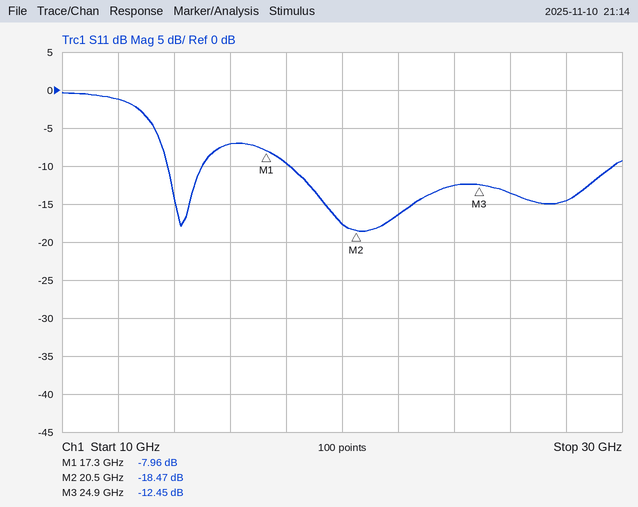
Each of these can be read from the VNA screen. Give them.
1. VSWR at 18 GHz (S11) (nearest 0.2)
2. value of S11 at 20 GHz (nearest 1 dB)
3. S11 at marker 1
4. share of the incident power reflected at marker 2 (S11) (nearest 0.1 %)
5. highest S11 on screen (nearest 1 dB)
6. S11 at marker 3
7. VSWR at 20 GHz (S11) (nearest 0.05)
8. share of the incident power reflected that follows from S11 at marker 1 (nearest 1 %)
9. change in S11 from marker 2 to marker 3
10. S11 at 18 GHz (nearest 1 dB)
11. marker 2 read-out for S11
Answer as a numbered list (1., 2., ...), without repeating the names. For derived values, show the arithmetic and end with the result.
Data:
1. |Γ| = 10^(-10/20) = 0.3162; VSWR = (1 + 0.3162)/(1 − 0.3162) ≈ 1.92, so 2.0 to the nearest 0.2
2. -18 dB
3. -7.96 dB
4. 10^(-18.47/10) ≈ 1.4 %
5. 0 dB
6. -12.45 dB
7. |Γ| = 10^(-18/20) = 0.1259; VSWR = (1 + 0.1259)/(1 − 0.1259) ≈ 1.29, so 1.30 to the nearest 0.05
8. 10^(-7.96/10) ≈ 16 %
9. -12.45 − (-18.47) = 6.02 dB
10. -10 dB
11. -18.47 dB
